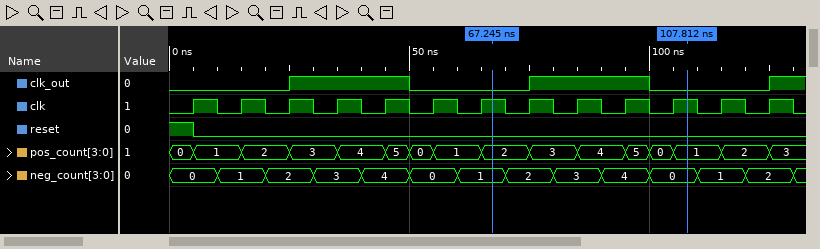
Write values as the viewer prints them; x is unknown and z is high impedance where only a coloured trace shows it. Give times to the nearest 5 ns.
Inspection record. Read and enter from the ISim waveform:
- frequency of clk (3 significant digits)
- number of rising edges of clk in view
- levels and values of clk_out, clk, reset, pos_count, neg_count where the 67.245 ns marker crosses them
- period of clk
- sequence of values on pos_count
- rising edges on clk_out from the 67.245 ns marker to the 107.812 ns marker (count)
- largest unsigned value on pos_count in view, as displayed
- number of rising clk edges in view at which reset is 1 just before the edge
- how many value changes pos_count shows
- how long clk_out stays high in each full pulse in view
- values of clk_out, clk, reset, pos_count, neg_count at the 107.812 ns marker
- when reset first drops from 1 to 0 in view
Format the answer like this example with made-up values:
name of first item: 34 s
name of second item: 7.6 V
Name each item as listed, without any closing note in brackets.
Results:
frequency of clk: 100 MHz
number of rising edges of clk in view: 13
levels and values of clk_out, clk, reset, pos_count, neg_count where the 67.245 ns marker crosses them: clk_out=0, clk=1, reset=0, pos_count=2, neg_count=1
period of clk: 10 ns
sequence of values on pos_count: 0, 1, 2, 3, 4, 5, 0, 1, 2, 3, 4, 5, 0, 1, 2, 3
rising edges on clk_out from the 67.245 ns marker to the 107.812 ns marker: 1
largest unsigned value on pos_count in view, as displayed: 5
number of rising clk edges in view at which reset is 1 just before the edge: 1
how many value changes pos_count shows: 15
how long clk_out stays high in each full pulse in view: 25 ns, 25 ns
values of clk_out, clk, reset, pos_count, neg_count at the 107.812 ns marker: clk_out=0, clk=1, reset=0, pos_count=1, neg_count=0
when reset first drops from 1 to 0 in view: 5 ns
